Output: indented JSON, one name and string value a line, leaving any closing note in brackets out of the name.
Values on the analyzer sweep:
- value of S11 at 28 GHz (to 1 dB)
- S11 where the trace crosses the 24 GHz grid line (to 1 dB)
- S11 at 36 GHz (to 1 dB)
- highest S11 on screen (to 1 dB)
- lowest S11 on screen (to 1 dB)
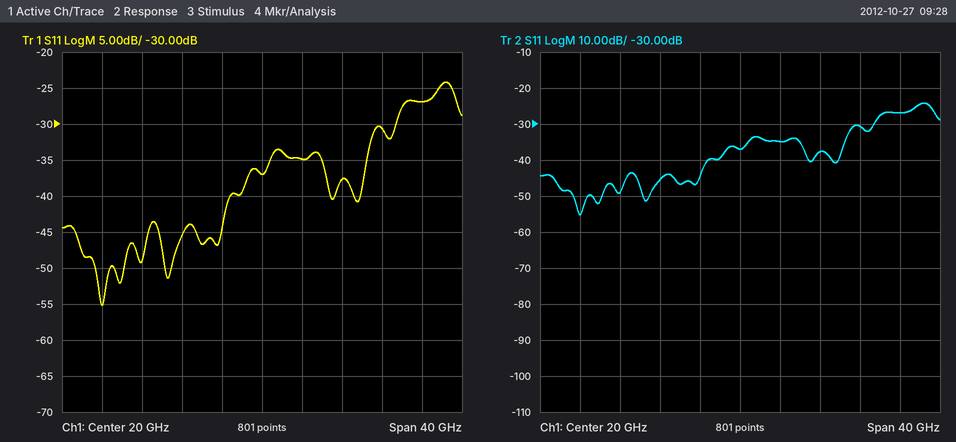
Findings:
{
  "value of S11 at 28 GHz": "-38 dB",
  "S11 where the trace crosses the 24 GHz grid line": "-35 dB",
  "S11 at 36 GHz": "-27 dB",
  "highest S11 on screen": "-24 dB",
  "lowest S11 on screen": "-55 dB"
}
